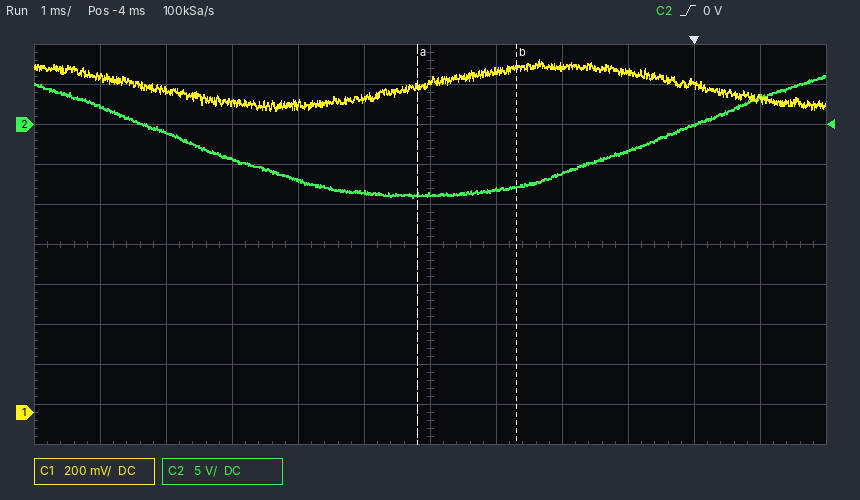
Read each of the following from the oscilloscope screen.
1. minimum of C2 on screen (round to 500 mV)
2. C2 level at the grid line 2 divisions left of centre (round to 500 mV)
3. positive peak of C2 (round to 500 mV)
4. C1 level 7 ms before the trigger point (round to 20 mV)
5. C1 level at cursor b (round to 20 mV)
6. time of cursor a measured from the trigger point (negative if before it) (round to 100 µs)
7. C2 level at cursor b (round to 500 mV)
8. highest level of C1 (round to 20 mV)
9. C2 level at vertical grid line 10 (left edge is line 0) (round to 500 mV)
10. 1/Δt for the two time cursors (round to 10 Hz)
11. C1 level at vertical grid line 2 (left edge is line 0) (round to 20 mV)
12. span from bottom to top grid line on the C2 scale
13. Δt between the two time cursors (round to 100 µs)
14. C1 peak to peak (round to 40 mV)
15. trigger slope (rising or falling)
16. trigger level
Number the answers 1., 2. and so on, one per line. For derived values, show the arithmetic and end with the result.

1. -9.0 V
2. -7.0 V
3. 6.0 V
4. 1.56 V
5. 1.72 V
6. -4.2 ms
7. -8.0 V
8. 1.76 V
9. 0.0 V
10. 1 / 1.5 ms ≈ 670 Hz
11. 1.62 V
12. 50 V
13. 1.5 ms
14. 240 mV
15. rising
16. 0 V
